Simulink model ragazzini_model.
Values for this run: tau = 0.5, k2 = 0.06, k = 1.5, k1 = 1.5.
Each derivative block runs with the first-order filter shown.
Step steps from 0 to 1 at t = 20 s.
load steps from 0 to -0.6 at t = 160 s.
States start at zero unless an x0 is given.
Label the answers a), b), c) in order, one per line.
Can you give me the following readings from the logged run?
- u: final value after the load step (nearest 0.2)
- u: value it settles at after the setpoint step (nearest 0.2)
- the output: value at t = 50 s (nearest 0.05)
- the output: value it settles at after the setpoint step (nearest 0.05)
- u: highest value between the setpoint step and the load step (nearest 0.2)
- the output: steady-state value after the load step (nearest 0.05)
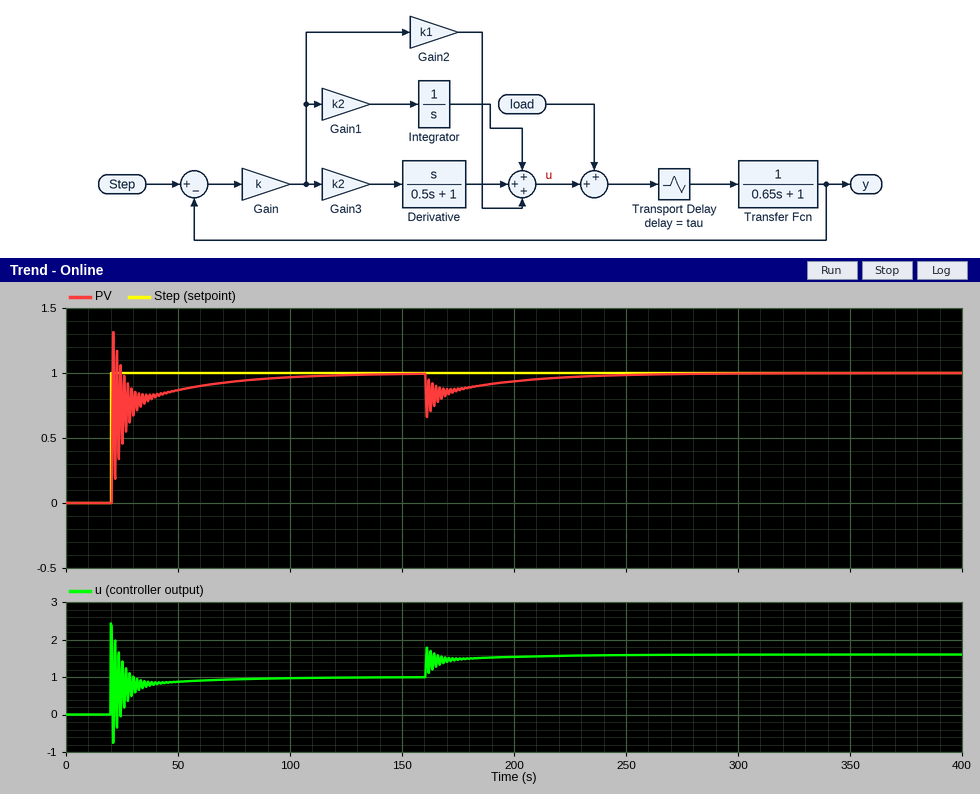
a) 1.6
b) 1.0
c) 0.85
d) 1.00
e) 2.4
f) 1.00
